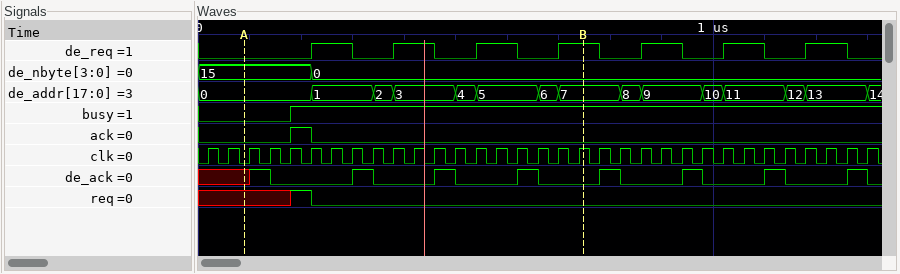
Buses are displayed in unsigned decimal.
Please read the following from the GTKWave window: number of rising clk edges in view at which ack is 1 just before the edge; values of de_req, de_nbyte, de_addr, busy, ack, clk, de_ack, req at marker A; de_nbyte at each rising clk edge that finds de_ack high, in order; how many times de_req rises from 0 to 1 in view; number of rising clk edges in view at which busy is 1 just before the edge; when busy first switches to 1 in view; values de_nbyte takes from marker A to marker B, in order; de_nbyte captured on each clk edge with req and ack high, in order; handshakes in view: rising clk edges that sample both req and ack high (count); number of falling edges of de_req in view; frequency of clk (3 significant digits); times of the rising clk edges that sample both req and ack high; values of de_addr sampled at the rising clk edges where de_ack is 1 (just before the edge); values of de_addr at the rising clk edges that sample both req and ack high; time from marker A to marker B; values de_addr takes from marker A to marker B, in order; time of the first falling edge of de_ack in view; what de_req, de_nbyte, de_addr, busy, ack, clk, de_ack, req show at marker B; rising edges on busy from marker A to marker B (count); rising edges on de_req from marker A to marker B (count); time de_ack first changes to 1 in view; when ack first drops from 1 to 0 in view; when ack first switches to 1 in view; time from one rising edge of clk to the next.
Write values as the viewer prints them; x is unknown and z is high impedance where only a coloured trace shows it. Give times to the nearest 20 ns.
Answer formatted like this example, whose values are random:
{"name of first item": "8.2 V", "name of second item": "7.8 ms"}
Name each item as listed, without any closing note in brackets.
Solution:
{"number of rising clk edges in view at which ack is 1 just before the edge": "1", "values of de_req, de_nbyte, de_addr, busy, ack, clk, de_ack, req at marker A": "de_req=0, de_nbyte=15, de_addr=0, busy=0, ack=0, clk=0, de_ack=x, req=x", "de_nbyte at each rising clk edge that finds de_ack high, in order": "15, 0, 0, 0, 0, 0, 0, 0", "how many times de_req rises from 0 to 1 in view": "7", "number of rising clk edges in view at which busy is 1 just before the edge": "28", "when busy first switches to 1 in view": "180 ns", "values de_nbyte takes from marker A to marker B, in order": "15, 0", "de_nbyte captured on each clk edge with req and ack high, in order": "15", "handshakes in view: rising clk edges that sample both req and ack high": "1", "number of falling edges of de_req in view": "7", "frequency of clk": "25.0 MHz", "times of the rising clk edges that sample both req and ack high": "220 ns", "values of de_addr sampled at the rising clk edges where de_ack is 1": "0, 1, 3, 5, 7, 9, 11, 13", "values of de_addr at the rising clk edges that sample both req and ack high": "0", "time from marker A to marker B": "660 ns", "values de_addr takes from marker A to marker B, in order": "0, 1, 2, 3, 4, 5, 6, 7", "time of the first falling edge of de_ack in view": "140 ns", "what de_req, de_nbyte, de_addr, busy, ack, clk, de_ack, req show at marker B": "de_req=1, de_nbyte=0, de_addr=7, busy=1, ack=0, clk=1, de_ack=0, req=0", "rising edges on busy from marker A to marker B": "1", "rising edges on de_req from marker A to marker B": "4", "time de_ack first changes to 1 in view": "100 ns", "when ack first drops from 1 to 0 in view": "220 ns", "when ack first switches to 1 in view": "180 ns", "time from one rising edge of clk to the next": "40 ns"}
